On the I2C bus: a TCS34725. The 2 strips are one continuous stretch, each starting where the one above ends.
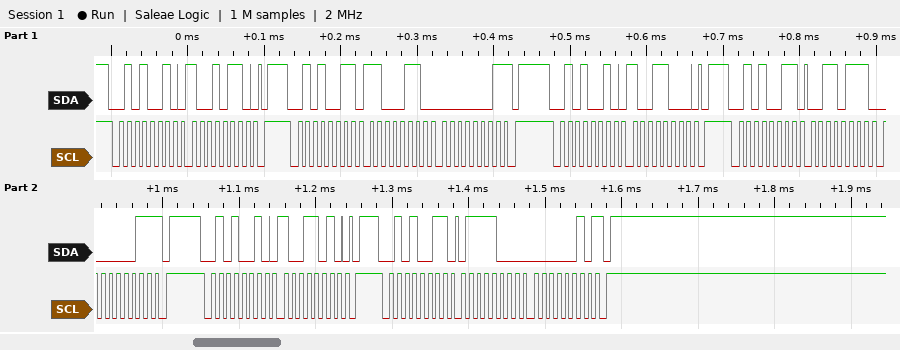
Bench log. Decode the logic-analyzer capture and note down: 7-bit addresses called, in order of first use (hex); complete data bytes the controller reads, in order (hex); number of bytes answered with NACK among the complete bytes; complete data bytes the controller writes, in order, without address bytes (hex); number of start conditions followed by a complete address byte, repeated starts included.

0x29
C6 01 37 03 78 02
3
96 98 9A
6
